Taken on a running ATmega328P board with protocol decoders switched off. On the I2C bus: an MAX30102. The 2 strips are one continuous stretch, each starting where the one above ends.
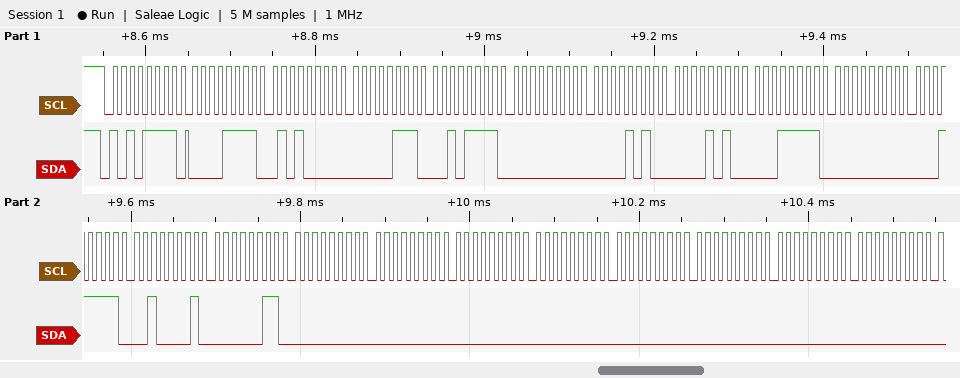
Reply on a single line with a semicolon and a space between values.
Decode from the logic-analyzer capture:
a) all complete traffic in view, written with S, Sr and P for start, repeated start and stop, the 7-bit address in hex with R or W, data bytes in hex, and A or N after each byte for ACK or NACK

S 57R A 0F A 50 A 07 A 2F A 00 A 0A A 0A A 1F A 00 A 1F A 21 A 03 A 00 A 00 A 00 A 00 A 00 A 00 A 00 A 00 A
